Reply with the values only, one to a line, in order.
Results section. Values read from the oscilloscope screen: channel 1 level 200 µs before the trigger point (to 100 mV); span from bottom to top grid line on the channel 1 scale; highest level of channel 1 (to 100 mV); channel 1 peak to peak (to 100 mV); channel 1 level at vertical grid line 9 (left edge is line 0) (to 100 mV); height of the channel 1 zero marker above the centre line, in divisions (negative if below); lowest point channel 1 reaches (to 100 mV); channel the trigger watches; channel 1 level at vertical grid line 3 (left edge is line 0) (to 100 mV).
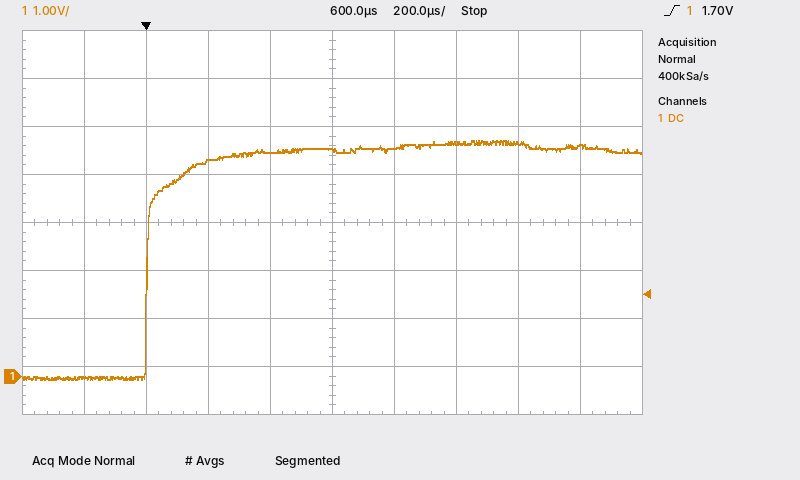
0.0 V
8 V
4.9 V
5.0 V
4.8 V
-3.2 div
-100 mV
channel 1
4.5 V
